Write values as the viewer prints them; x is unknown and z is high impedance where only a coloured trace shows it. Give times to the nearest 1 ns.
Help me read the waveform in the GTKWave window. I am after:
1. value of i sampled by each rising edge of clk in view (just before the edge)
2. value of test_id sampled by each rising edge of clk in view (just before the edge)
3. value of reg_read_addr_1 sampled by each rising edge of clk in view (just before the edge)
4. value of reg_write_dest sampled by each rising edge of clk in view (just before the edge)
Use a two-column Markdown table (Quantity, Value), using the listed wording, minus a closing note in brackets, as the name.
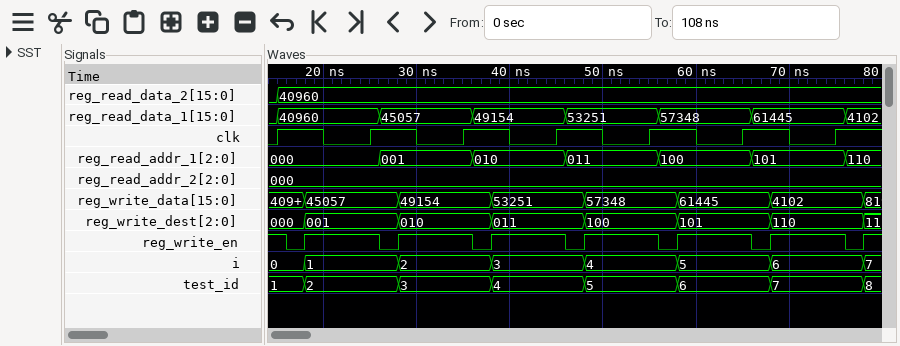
| Quantity | Value |
|---|---|
| value of i sampled by each rising edge of clk in view | 0, 1, 2, 3, 4, 5, 6 |
| value of test_id sampled by each rising edge of clk in view | 1, 2, 3, 4, 5, 6, 7 |
| value of reg_read_addr_1 sampled by each rising edge of clk in view | 000, 000, 001, 010, 011, 100, 101 |
| value of reg_write_dest sampled by each rising edge of clk in view | 000, 001, 010, 011, 100, 101, 110 |
